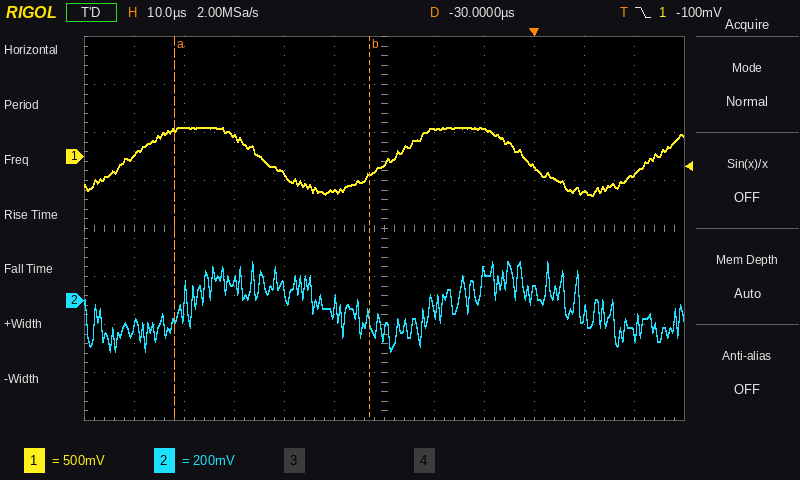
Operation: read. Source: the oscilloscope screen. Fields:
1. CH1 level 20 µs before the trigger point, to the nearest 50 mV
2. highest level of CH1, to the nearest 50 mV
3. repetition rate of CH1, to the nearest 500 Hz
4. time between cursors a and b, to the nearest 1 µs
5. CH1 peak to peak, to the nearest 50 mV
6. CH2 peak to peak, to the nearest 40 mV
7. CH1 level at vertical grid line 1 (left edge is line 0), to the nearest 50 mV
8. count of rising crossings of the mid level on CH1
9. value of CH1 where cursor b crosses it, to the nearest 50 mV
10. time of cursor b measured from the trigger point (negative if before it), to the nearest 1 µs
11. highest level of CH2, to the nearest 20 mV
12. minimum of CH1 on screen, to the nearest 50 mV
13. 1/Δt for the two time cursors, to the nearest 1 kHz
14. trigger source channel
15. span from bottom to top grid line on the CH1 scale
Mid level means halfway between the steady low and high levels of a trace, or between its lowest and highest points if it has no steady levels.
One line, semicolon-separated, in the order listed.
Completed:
300 mV; 300 mV; 19.0 kHz; 39 µs; 700 mV; 360 mV; 0 mV; 3; -200 mV; -33 µs; 160 mV; -400 mV; 26 kHz; CH1; 4 V
